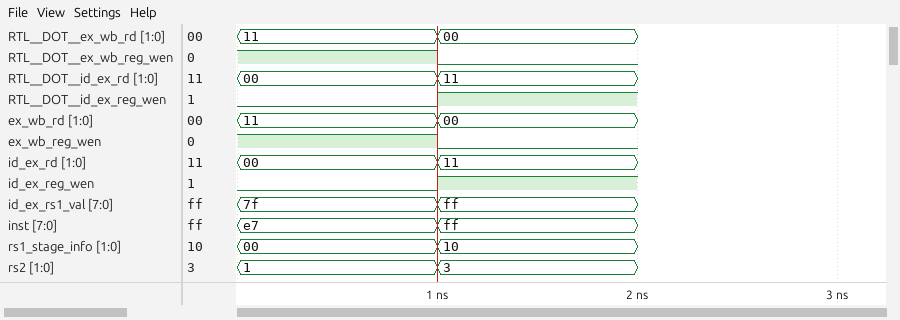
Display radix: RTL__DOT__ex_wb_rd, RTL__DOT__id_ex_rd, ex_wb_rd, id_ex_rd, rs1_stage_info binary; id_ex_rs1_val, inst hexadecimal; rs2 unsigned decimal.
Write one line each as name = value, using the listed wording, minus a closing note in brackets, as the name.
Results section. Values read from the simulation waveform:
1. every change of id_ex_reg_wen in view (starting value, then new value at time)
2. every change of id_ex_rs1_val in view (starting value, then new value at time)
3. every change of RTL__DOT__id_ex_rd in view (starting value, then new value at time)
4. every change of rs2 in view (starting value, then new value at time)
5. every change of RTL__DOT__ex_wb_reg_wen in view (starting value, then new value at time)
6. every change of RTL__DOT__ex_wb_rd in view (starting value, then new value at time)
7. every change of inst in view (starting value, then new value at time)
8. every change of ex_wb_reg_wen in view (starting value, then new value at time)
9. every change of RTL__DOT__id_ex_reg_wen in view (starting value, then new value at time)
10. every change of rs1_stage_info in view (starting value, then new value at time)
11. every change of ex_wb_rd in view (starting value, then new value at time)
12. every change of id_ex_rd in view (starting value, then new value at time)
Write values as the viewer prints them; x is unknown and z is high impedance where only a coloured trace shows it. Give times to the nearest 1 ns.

every change of id_ex_reg_wen in view = 0, 1 at 1 ns
every change of id_ex_rs1_val in view = 7f, ff at 1 ns
every change of RTL__DOT__id_ex_rd in view = 00, 11 at 1 ns
every change of rs2 in view = 1, 3 at 1 ns
every change of RTL__DOT__ex_wb_reg_wen in view = 1, 0 at 1 ns
every change of RTL__DOT__ex_wb_rd in view = 11, 00 at 1 ns
every change of inst in view = e7, ff at 1 ns
every change of ex_wb_reg_wen in view = 1, 0 at 1 ns
every change of RTL__DOT__id_ex_reg_wen in view = 0, 1 at 1 ns
every change of rs1_stage_info in view = 00, 10 at 1 ns
every change of ex_wb_rd in view = 11, 00 at 1 ns
every change of id_ex_rd in view = 00, 11 at 1 ns
